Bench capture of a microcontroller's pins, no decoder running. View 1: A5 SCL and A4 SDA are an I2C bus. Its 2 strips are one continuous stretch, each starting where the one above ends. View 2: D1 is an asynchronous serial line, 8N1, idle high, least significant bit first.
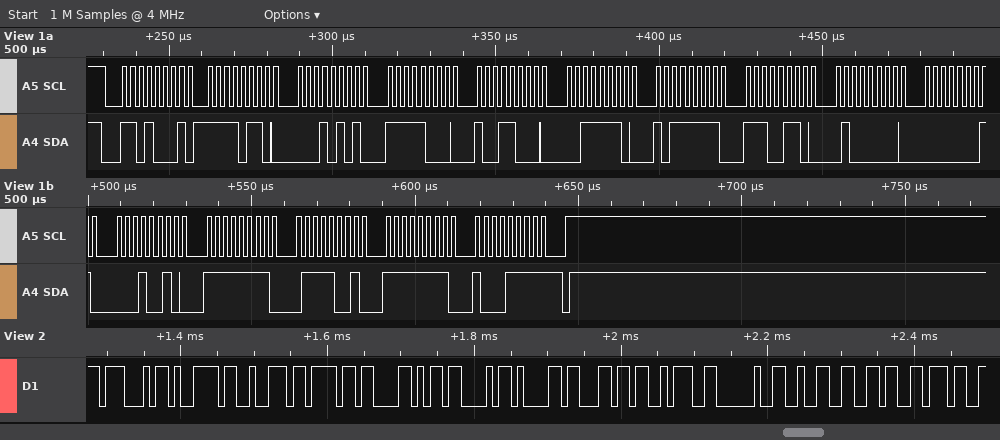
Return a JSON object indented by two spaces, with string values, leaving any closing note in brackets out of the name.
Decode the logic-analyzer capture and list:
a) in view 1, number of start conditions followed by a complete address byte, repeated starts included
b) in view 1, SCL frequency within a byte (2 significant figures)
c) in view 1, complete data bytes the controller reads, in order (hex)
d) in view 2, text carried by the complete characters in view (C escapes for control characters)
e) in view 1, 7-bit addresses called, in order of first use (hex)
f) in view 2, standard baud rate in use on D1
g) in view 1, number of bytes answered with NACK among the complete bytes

{
  "in view 1, number of start conditions followed by a complete address byte, repeated starts included": "1",
  "in view 1, SCL frequency within a byte": "400 kHz",
  "in view 1, complete data bytes the controller reads, in order": "F6 15 F8 98 3E BF E6 40 01 12 FF 79 FF 8F",
  "in view 2, text carried by the complete characters in view": "\"GyroXCal: 267\"",
  "in view 1, 7-bit addresses called, in order of first use": "0x68",
  "in view 2, standard baud rate in use on D1": "115200 baud",
  "in view 1, number of bytes answered with NACK among the complete bytes": "1"
}
